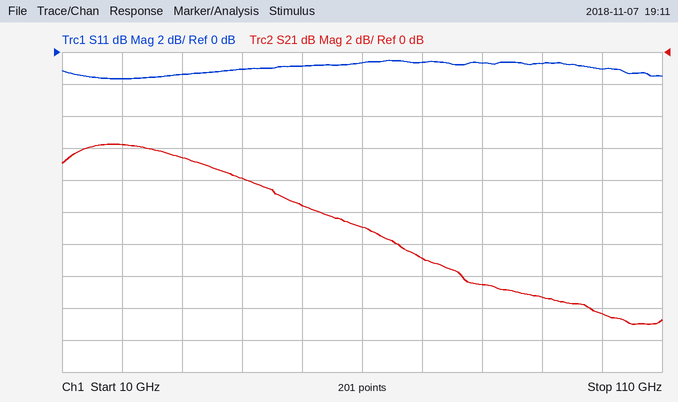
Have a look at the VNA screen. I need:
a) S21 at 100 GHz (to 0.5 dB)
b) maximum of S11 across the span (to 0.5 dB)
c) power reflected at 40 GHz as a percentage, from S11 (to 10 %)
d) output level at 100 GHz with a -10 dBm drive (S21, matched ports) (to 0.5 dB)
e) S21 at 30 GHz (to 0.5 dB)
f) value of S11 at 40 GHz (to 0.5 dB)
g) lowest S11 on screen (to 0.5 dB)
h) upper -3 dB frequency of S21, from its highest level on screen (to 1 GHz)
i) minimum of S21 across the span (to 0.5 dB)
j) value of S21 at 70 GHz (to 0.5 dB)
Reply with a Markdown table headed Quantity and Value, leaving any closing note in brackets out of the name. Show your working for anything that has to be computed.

| Quantity | Value |
|---|---|
| S21 at 100 GHz | -16.5 dB |
| maximum of S11 across the span | -0.5 dB |
| power reflected at 40 GHz as a percentage, from S11 | 10^(-1/10) ≈ 79.4 %, so 80 % to the nearest 10 % |
| output level at 100 GHz with a -10 dBm drive (S21, matched ports) | -10 dBm + (-16.5 dB) = -26.5 dBm |
| S21 at 30 GHz | -6.5 dB |
| value of S11 at 40 GHz | -1.0 dB |
| lowest S11 on screen | -1.5 dB |
| upper -3 dB frequency of S21, from its highest level on screen | 45 GHz |
| minimum of S21 across the span | -17.0 dB |
| value of S21 at 70 GHz | -13.0 dB |
